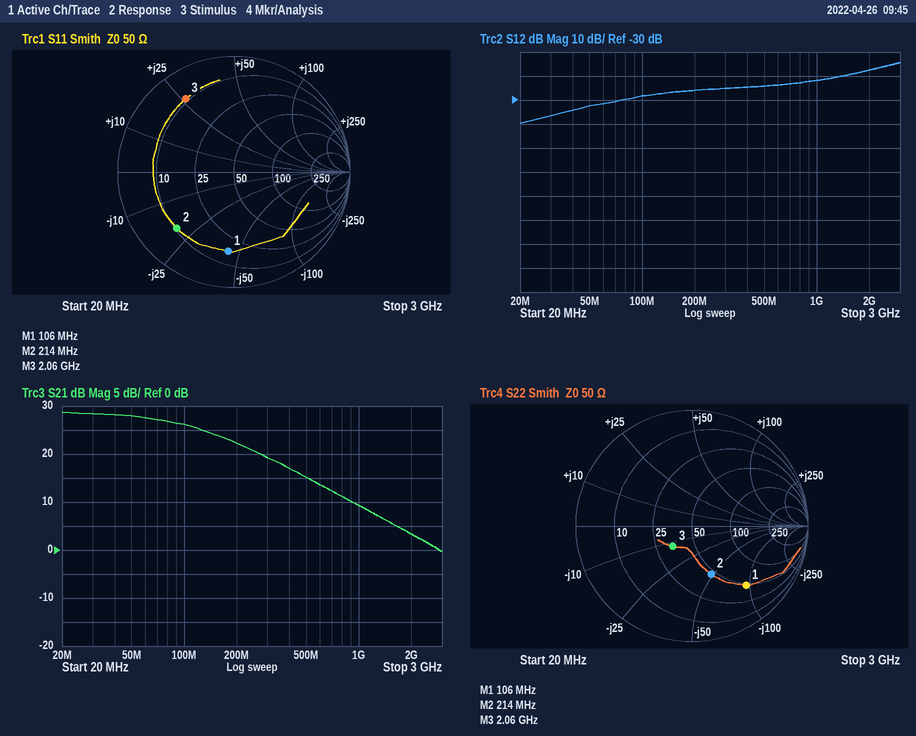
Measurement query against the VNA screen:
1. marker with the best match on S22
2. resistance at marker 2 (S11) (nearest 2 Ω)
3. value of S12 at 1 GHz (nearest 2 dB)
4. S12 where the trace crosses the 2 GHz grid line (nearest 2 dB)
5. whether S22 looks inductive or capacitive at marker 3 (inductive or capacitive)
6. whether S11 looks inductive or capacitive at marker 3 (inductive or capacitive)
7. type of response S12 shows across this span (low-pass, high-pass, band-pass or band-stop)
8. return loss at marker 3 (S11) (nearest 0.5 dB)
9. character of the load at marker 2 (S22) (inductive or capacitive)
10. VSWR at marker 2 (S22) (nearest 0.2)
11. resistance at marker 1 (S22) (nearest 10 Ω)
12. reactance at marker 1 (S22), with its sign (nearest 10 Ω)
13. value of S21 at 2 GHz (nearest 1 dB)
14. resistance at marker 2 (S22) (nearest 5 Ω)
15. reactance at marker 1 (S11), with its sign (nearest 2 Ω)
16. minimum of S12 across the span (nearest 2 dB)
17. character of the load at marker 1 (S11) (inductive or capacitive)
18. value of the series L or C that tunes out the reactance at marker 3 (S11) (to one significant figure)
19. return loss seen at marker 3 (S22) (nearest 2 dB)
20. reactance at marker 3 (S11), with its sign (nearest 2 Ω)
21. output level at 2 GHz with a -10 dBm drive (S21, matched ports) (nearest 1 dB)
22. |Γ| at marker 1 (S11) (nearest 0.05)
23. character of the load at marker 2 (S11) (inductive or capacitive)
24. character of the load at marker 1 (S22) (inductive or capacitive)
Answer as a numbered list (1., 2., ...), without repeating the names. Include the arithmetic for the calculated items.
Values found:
1. marker 3
2. 10 Ω
3. -22 dB
4. -18 dB
5. capacitive
6. inductive
7. high-pass
8. 2.5 dB
9. capacitive
10. 2.6
11. 50 Ω
12. -90 Ω
13. 3 dB
14. 45 Ω
15. -44 Ω
16. -40 dB
17. capacitive
18. C = 1/(2π × 2.06 GHz × 26 Ω) ≈ 3 pF
19. 12 dB
20. +26 Ω
21. -10 dBm + (3 dB) = -7 dBm
22. 0.70
23. capacitive
24. capacitive
